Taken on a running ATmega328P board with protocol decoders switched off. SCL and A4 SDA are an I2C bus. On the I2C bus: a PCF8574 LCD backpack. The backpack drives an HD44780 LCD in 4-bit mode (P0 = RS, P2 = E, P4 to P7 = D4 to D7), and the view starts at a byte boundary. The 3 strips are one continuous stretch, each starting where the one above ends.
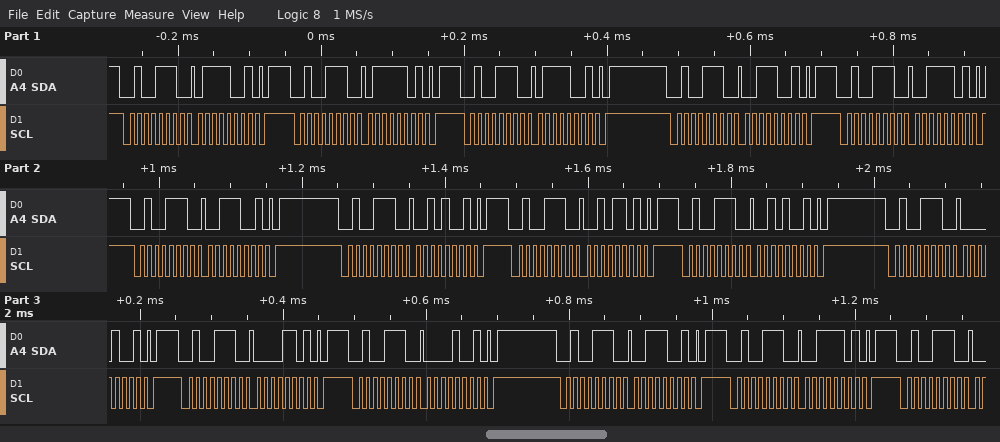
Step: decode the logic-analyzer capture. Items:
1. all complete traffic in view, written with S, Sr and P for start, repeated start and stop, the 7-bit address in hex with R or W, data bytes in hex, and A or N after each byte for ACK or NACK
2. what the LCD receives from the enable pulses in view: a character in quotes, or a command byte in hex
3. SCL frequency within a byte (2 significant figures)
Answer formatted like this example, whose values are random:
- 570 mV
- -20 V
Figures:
- S 27W A 79 A P S 27W A 7D A P S 27W A 79 A P S 27W A 39 A P S 27W A 3D A P S 27W A 39 A P S 27W A 29 A P S 27W A 2D A P S 27W A 29 A P S 27W A 09 A P S 27W A 0D A P S 27W A 09 A P S 27W A 39 A P S 27W A 3D A P S 27W A
- 's' ' '
- 100 kHz
